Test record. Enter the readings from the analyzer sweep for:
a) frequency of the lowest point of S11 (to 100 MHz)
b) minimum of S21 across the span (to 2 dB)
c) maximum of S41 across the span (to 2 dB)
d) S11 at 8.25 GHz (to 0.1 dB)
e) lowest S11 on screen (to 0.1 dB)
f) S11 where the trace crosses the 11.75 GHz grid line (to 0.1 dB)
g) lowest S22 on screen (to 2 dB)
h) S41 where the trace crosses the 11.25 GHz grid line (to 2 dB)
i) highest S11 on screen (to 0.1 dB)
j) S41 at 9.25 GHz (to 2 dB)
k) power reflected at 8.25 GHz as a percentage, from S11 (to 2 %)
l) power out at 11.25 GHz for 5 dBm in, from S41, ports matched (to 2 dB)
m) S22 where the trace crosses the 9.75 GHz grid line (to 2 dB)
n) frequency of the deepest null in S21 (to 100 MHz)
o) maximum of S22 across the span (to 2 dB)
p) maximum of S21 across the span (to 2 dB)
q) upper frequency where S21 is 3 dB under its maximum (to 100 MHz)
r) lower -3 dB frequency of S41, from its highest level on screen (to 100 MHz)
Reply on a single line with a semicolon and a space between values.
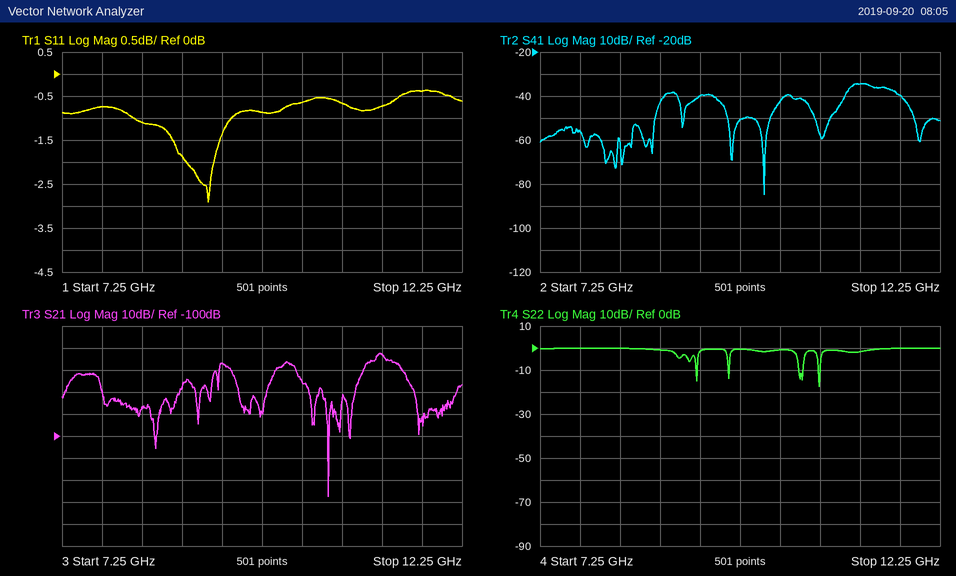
9.1 GHz; -128 dB; -34 dB; -1.1 dB; -2.9 dB; -0.4 dB; -18 dB; -34 dB; -0.4 dB; -40 dB; 78 %; -30 dBm; 0 dB; 10.6 GHz; 0 dB; -62 dB; 11.3 GHz; 11.1 GHz
